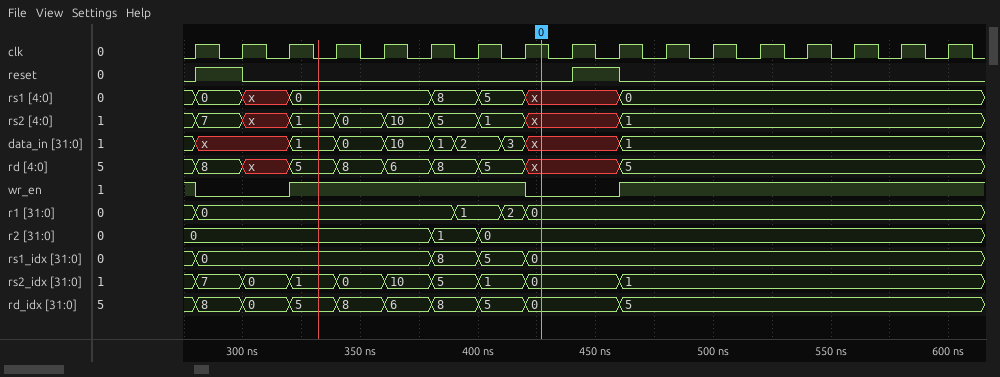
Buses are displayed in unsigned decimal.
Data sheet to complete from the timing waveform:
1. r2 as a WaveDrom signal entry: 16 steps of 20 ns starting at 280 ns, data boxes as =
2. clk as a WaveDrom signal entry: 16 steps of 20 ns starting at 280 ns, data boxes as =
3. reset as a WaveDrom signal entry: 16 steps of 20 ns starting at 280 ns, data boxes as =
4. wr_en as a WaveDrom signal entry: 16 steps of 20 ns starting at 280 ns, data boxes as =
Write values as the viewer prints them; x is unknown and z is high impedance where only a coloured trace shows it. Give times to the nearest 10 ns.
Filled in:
{name: 'r2', wave: '=....==.........', data: '0 1 0'}
{name: 'clk', wave: 'p...............'}
{name: 'reset', wave: '10......10......'}
{name: 'wr_en', wave: '0.1....0.1......'}
